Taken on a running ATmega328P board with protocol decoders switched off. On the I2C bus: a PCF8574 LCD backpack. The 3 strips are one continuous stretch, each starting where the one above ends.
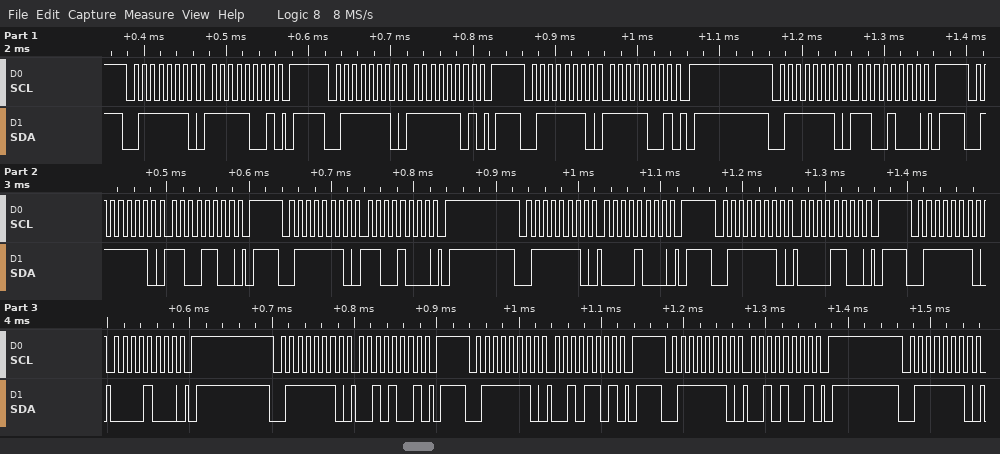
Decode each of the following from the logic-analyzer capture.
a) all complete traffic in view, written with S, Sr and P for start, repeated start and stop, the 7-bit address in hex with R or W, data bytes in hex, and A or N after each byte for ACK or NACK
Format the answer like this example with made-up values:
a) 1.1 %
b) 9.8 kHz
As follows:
a) S 3FW A F9 A P S 3FW A FD A P S 3FW A F9 A P S 3FW A C8 A P S 3FW A CC A P S 3FW A C8 A P S 3FW A 08 A P S 3FW A 0C A P S 3FW A 08 A P S 3FW A 29 A P S 3FW A 2D A P S 3FW A 29 A P S 3FW A
